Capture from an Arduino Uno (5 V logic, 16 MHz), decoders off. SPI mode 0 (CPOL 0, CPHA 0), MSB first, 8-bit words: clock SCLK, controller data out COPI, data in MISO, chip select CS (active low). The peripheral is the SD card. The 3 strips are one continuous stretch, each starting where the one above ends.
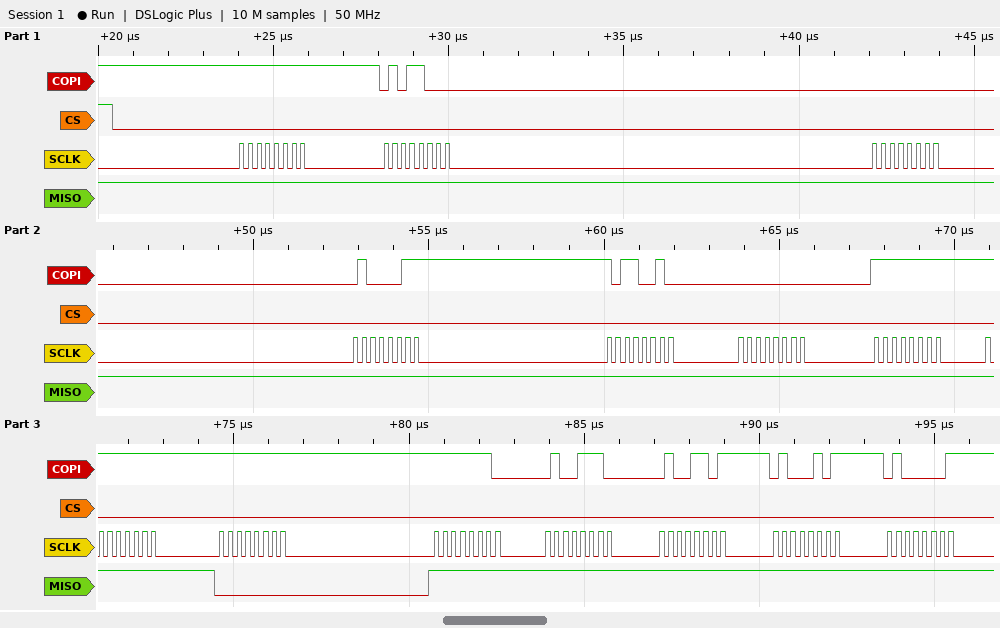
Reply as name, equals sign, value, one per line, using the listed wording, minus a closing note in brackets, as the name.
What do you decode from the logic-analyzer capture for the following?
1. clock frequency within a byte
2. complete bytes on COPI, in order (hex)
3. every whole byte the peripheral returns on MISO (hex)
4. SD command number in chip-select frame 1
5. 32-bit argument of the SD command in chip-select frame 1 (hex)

clock frequency within a byte = 4 MHz
complete bytes on COPI, in order = FF 58 00 43 B2 00 FF FF FF FE 4E 4D 45 41
every whole byte the peripheral returns on MISO = FF FF FF FF FF FF FF FF 00 FF FF FF FF FF
SD command number in chip-select frame 1 = CMD24
32-bit argument of the SD command in chip-select frame 1 = 0x0043B200
